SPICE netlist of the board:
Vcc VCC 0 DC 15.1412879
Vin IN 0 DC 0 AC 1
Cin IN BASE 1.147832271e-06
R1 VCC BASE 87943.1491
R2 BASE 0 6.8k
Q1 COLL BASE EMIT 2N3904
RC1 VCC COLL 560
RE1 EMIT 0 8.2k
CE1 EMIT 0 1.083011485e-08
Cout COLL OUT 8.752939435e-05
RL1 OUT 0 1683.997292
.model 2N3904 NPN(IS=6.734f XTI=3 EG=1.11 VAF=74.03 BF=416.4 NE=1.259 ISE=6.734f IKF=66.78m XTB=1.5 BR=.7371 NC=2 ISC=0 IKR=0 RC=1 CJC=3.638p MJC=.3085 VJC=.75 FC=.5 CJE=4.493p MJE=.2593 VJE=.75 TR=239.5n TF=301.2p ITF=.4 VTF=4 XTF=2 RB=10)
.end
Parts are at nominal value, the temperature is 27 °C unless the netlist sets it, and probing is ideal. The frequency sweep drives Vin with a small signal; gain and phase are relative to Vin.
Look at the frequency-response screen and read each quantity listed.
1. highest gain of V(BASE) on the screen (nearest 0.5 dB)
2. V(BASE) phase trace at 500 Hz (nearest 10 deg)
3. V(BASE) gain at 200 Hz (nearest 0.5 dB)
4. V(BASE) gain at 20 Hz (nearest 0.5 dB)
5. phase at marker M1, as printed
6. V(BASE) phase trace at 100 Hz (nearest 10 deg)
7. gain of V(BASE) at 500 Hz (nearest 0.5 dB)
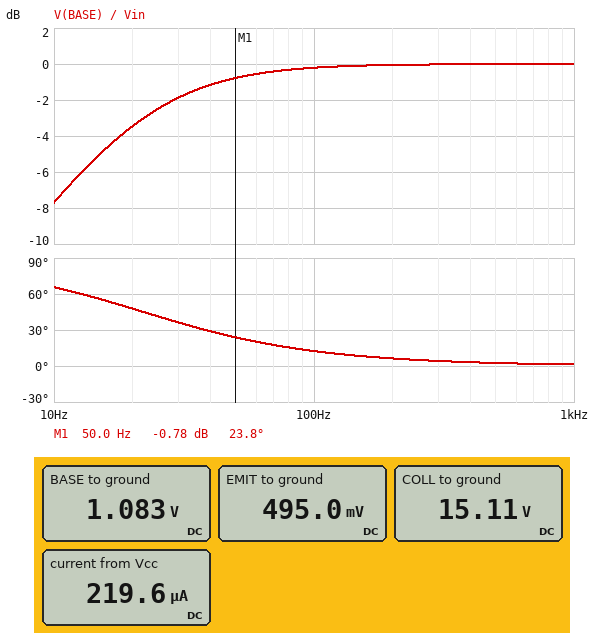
0 dB
0 deg
0 dB
-3.5 dB
23.8 deg
10 deg
0 dB
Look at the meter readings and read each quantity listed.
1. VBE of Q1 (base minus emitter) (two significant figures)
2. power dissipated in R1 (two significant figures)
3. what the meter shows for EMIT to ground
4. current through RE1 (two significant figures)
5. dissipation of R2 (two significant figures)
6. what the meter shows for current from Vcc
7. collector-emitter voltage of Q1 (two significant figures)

590 mV
2.2 mW
495.0 mV
60 µA
170 µW
219.6 µA
15 V
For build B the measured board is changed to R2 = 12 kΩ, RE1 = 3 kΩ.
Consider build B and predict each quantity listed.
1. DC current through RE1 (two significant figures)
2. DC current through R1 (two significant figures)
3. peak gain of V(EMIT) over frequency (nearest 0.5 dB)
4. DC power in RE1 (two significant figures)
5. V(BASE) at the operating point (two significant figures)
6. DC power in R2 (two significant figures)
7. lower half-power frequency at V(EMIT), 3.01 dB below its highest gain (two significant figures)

380 µA
150 µA
0 dB
440 µW
1.8 V
270 µW
13 Hz
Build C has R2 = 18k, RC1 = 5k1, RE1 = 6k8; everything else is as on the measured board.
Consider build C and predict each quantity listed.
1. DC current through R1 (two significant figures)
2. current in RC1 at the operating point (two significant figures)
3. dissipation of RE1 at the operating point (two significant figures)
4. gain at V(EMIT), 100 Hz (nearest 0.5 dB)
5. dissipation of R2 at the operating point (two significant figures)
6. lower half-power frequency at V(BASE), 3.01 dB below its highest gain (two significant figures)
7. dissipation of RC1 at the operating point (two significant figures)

140 µA
280 µA
540 µW
0 dB
360 µW
9.4 Hz
400 µW
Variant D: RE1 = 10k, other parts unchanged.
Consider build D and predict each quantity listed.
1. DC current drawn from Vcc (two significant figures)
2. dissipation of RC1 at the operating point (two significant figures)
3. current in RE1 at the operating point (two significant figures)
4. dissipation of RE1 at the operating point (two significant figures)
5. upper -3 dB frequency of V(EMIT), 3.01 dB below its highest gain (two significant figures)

210 µA
1.4 µW
50 µA
25 µW
30 kHz
